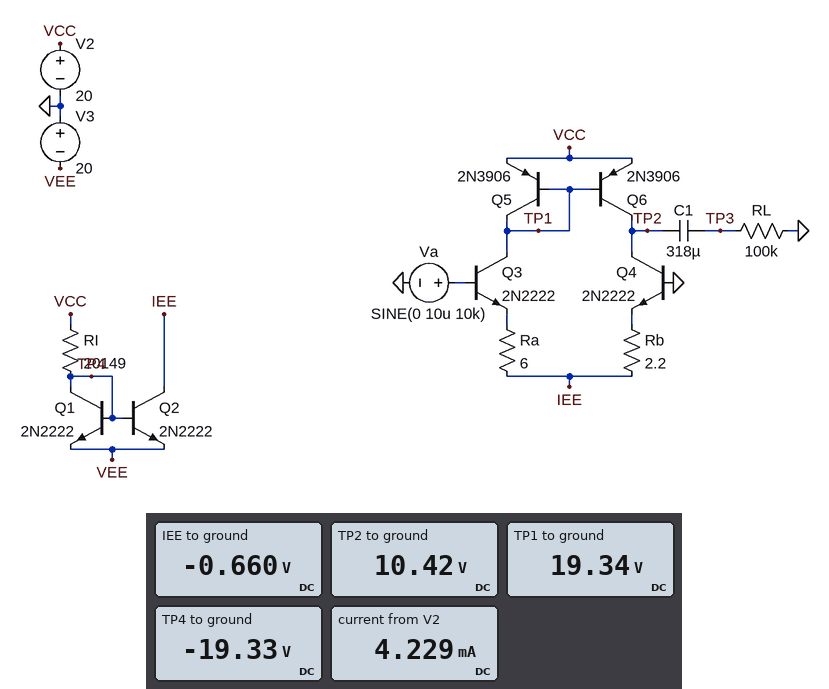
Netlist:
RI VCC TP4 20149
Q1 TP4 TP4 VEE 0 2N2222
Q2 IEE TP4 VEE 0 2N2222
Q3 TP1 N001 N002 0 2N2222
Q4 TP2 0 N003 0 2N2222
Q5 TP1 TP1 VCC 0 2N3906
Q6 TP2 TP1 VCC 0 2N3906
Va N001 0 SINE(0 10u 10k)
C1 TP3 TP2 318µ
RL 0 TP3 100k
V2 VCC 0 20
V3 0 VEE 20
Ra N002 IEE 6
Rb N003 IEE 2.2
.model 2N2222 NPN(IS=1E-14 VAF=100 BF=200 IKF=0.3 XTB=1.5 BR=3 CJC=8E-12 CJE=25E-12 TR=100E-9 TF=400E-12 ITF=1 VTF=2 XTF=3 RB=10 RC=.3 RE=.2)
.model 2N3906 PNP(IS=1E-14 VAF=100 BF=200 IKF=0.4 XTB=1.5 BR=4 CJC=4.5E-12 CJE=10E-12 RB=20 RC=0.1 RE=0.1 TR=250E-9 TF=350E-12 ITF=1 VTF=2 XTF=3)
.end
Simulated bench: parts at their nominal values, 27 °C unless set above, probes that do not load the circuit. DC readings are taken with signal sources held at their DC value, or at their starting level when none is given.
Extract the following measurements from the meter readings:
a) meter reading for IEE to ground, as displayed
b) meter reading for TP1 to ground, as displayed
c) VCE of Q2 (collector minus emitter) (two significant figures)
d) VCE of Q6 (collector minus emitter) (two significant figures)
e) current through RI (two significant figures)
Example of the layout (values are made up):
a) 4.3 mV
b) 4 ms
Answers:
a) -0.660 V
b) 19.34 V
c) 19 V
d) -9.6 V
e) 2.0 mA
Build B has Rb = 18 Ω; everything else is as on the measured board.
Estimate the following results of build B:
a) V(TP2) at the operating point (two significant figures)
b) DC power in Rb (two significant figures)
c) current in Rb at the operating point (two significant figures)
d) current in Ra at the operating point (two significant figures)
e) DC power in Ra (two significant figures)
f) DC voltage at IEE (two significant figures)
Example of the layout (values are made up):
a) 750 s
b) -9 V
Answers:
a) 20 V
b) 16 µW
c) 950 µA
d) 1.3 mA
e) 11 µW
f) -670 mV
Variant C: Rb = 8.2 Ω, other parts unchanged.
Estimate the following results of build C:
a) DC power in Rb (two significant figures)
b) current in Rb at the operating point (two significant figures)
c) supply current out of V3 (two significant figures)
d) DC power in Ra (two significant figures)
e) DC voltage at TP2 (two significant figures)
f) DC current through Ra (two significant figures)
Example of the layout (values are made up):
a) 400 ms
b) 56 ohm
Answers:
a) 10 µW
b) 1.1 mA
c) 4.2 mA
d) 8.4 µW
e) 20 V
f) 1.2 mA
